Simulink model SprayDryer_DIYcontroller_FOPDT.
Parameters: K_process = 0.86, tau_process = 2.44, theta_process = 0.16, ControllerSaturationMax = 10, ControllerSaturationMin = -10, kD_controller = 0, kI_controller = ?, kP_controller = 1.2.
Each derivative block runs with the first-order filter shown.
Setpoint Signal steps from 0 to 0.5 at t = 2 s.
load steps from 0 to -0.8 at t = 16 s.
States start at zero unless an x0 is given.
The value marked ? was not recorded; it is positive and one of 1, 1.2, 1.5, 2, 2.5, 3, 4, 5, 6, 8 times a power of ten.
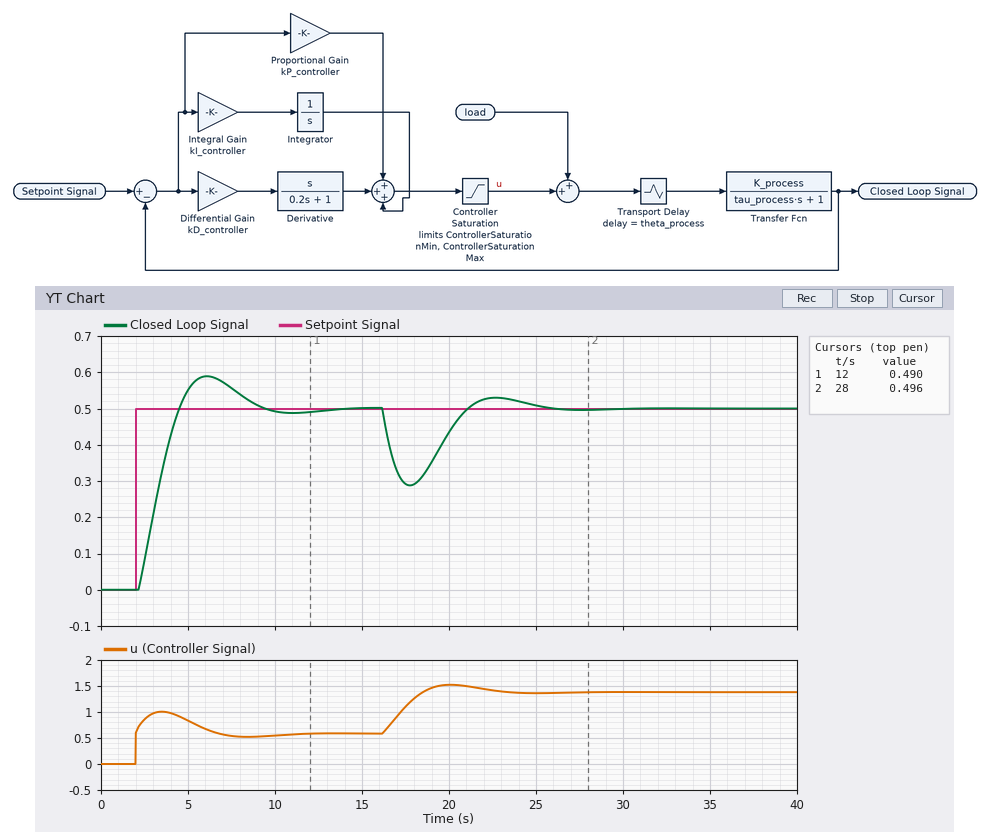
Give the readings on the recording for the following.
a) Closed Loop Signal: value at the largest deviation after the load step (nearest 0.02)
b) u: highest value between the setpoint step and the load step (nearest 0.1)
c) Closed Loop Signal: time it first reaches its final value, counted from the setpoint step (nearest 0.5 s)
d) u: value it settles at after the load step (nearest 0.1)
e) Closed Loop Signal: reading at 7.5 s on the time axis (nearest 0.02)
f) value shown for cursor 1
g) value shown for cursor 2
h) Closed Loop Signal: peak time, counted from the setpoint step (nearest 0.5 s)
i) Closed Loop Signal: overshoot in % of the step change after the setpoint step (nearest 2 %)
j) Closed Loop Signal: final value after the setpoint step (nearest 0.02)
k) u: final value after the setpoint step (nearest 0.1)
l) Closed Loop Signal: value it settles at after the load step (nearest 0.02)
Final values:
0.28
1.0
2.5 s
1.4
0.56
0.490
0.496
4.0 s
18 %
0.50
0.6
0.50
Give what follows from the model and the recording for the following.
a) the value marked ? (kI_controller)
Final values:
1.5
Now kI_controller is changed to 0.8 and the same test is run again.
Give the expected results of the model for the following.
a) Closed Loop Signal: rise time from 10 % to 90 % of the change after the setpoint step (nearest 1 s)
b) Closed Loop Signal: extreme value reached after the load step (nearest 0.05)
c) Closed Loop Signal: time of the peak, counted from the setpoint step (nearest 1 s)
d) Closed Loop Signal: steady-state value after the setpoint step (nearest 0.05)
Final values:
3 s
0.25
6 s
0.50
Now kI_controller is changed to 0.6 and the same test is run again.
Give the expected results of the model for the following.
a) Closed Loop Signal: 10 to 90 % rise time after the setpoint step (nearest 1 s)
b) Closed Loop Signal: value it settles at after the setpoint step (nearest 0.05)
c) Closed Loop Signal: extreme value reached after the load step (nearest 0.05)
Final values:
4 s
0.50
0.25
